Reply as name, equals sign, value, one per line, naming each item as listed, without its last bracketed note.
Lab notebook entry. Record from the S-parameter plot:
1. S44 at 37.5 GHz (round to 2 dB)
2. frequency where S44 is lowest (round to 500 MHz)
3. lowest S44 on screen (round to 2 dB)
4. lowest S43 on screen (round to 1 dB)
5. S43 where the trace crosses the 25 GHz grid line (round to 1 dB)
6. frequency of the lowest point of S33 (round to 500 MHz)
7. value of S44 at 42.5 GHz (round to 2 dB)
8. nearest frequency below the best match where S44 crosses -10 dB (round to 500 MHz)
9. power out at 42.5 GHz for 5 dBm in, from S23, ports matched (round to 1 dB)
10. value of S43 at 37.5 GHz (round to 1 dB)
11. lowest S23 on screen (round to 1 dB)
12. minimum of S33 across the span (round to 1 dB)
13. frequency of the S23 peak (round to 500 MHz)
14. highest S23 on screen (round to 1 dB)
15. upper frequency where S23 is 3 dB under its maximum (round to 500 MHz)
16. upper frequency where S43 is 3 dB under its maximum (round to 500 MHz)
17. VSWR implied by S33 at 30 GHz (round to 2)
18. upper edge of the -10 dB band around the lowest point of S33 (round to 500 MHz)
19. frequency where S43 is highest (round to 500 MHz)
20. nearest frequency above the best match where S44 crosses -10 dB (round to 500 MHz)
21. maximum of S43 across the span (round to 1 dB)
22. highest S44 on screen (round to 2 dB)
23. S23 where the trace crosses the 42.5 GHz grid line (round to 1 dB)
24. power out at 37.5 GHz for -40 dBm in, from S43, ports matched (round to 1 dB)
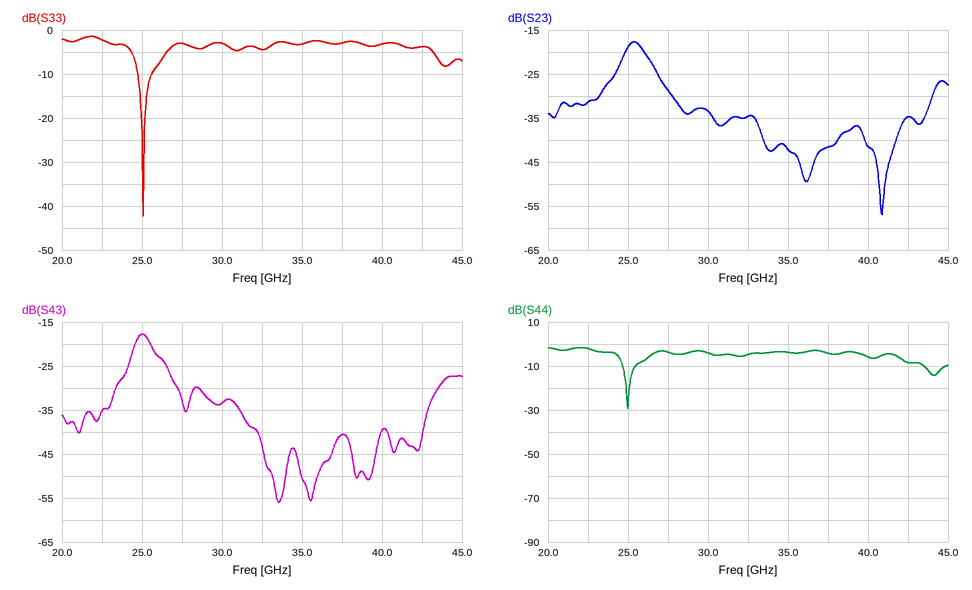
S44 at 37.5 GHz = -4 dB
frequency where S44 is lowest = 25.0 GHz
lowest S44 on screen = -30 dB
lowest S43 on screen = -56 dB
S43 where the trace crosses the 25 GHz grid line = -18 dB
frequency of the lowest point of S33 = 25.0 GHz
value of S44 at 42.5 GHz = -8 dB
nearest frequency below the best match where S44 crosses -10 dB = 24.5 GHz
power out at 42.5 GHz for 5 dBm in, from S23, ports matched = -30 dBm
value of S43 at 37.5 GHz = -41 dB
lowest S23 on screen = -57 dB
minimum of S33 across the span = -42 dB
frequency of the S23 peak = 25.5 GHz
highest S23 on screen = -18 dB
upper frequency where S23 is 3 dB under its maximum = 26.0 GHz
upper frequency where S43 is 3 dB under its maximum = 25.5 GHz
VSWR implied by S33 at 30 GHz = 6
upper edge of the -10 dB band around the lowest point of S33 = 25.5 GHz
frequency where S43 is highest = 25.0 GHz
nearest frequency above the best match where S44 crosses -10 dB = 25.5 GHz
maximum of S43 across the span = -18 dB
highest S44 on screen = -2 dB
S23 where the trace crosses the 42.5 GHz grid line = -35 dB
power out at 37.5 GHz for -40 dBm in, from S43, ports matched = -81 dBm
